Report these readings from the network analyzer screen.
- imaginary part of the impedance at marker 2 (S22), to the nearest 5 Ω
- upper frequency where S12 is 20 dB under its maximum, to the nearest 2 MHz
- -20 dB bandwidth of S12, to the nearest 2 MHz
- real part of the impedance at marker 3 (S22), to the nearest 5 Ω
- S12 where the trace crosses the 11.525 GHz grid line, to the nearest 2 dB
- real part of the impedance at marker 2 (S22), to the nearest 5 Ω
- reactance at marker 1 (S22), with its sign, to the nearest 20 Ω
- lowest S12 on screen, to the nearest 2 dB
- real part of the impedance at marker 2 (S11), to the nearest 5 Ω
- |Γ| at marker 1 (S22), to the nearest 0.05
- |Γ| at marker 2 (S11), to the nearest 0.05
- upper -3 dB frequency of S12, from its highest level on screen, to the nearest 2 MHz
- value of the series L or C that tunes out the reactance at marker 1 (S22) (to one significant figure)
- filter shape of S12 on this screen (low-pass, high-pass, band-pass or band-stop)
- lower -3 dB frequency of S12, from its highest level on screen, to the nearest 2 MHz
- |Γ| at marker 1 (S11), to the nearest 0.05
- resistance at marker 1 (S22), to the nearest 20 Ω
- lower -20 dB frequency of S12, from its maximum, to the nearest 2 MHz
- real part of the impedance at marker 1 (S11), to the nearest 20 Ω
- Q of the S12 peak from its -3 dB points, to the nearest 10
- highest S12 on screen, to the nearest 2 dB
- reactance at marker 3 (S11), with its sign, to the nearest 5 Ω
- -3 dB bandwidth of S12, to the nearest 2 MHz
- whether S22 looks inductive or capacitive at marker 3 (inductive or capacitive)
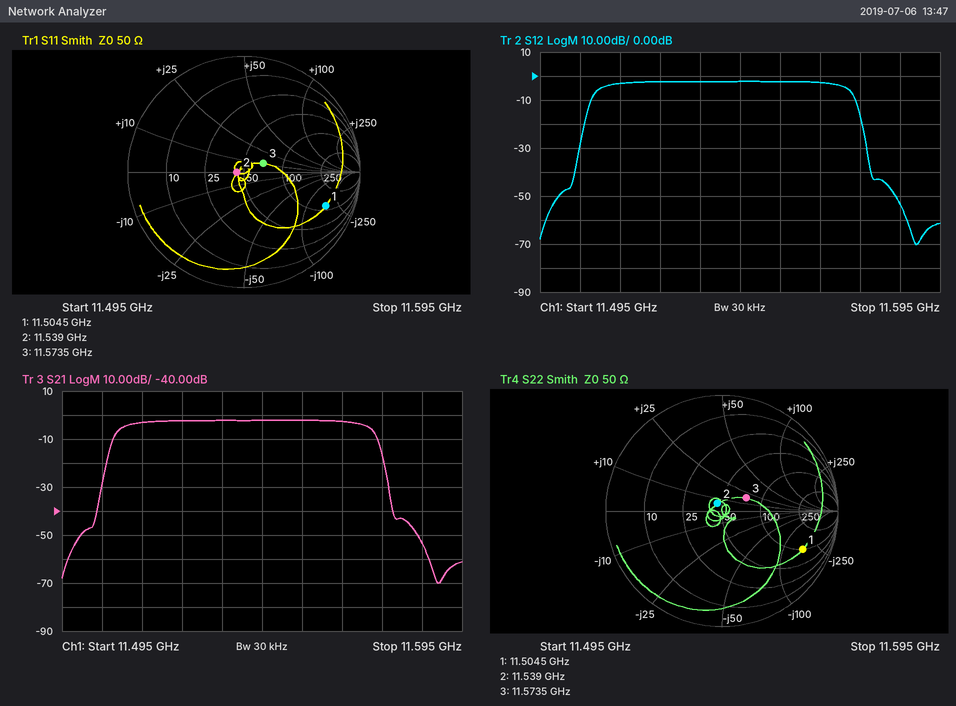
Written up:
+5 Ω
11.576 GHz
70 MHz
75 Ω
-2 dB
45 Ω
-160 Ω
-70 dB
45 Ω
0.75
0.05
11.572 GHz
2 nH
band-pass
11.510 GHz
0.75
100 Ω
11.506 GHz
120 Ω
190
-2 dB
+10 Ω
62 MHz
inductive
